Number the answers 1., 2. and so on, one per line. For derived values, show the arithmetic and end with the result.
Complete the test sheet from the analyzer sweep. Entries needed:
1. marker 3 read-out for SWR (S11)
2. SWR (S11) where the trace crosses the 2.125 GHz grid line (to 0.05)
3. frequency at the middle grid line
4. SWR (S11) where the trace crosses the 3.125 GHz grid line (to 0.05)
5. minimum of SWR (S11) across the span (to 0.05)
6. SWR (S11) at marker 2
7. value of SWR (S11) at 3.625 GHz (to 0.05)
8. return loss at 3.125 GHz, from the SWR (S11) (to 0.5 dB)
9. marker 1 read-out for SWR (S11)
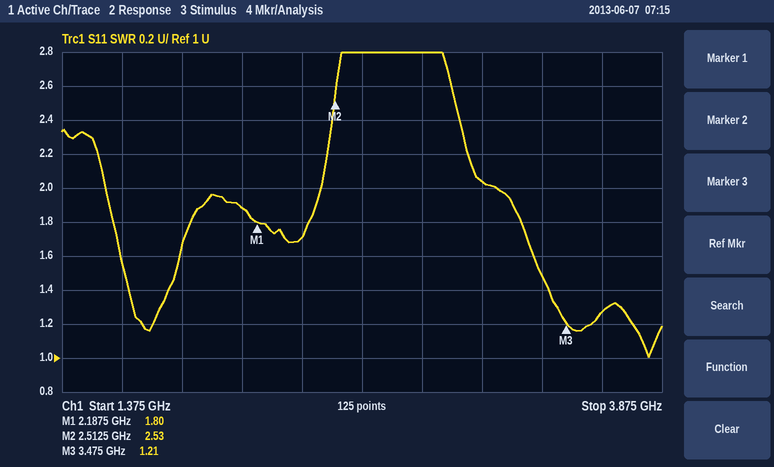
1. 1.21
2. 1.90
3. 2.625 GHz
4. 2.05
5. 1.00
6. 2.53
7. 1.25
8. −20 log10((2.05 − 1)/(2.05 + 1)) ≈ 9.26 dB, so 9.5 dB to the nearest 0.5 dB
9. 1.80
